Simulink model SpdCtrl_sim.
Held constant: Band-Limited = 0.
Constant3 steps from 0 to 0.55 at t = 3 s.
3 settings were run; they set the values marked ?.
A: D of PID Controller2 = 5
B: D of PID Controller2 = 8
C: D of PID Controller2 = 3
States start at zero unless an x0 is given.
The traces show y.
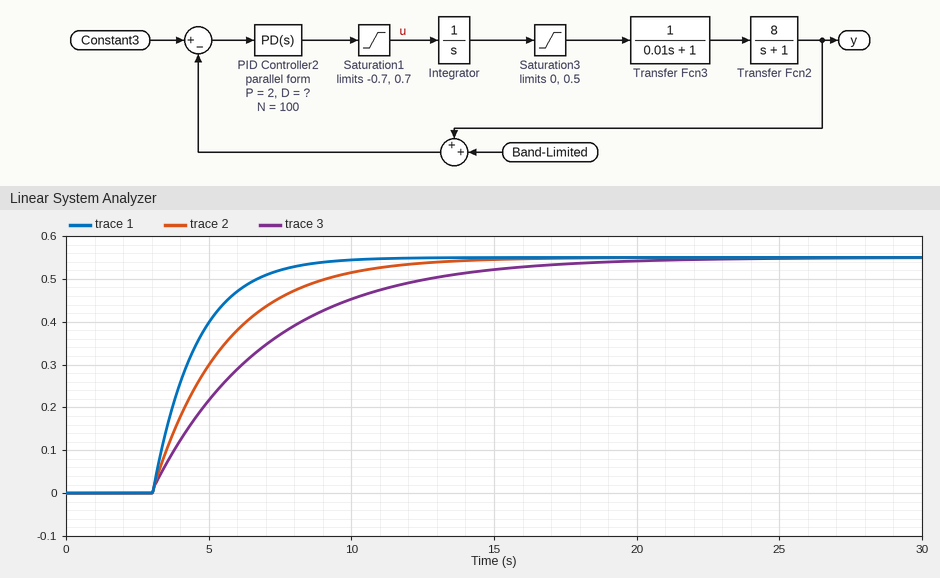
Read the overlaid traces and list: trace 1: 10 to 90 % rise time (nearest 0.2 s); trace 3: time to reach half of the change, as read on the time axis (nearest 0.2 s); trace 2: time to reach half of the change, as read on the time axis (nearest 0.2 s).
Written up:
3.4 s
5.8 s
4.8 s
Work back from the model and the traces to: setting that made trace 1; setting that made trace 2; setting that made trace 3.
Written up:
C
A
B
